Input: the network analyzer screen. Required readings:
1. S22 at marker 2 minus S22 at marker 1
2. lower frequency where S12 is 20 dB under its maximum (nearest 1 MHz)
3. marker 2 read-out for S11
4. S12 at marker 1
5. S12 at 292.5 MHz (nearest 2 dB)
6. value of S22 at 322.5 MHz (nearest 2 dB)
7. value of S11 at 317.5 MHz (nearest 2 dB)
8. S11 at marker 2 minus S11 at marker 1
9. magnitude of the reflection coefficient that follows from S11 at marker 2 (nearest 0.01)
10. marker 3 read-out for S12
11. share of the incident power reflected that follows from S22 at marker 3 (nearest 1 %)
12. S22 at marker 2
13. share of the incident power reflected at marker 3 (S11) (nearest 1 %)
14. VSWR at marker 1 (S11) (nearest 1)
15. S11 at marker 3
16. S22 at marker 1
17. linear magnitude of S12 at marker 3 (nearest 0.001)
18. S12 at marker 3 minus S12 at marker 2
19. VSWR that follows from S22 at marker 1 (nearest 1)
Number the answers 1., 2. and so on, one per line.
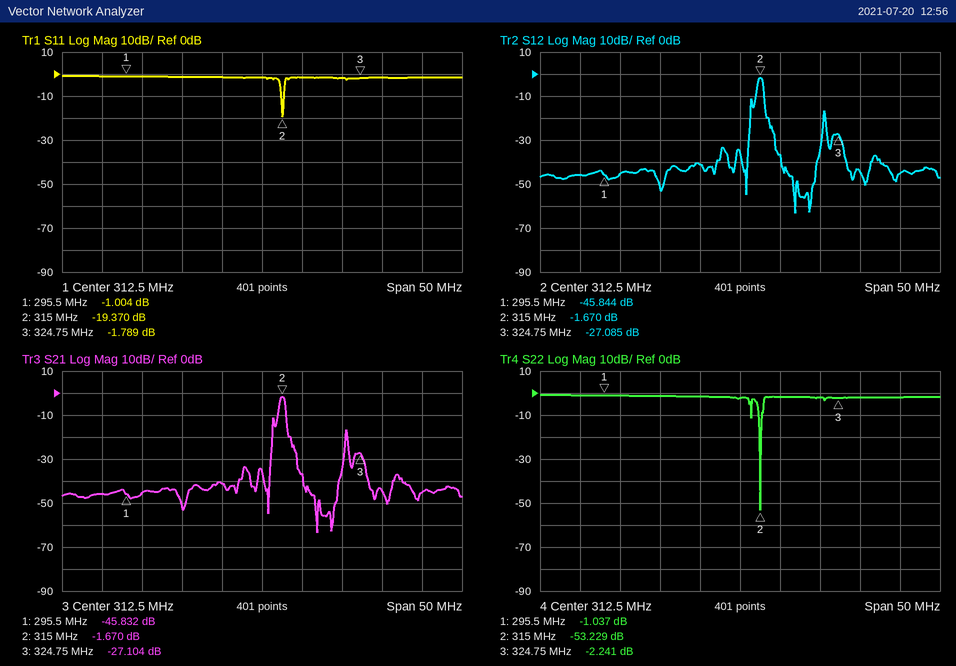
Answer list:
1. -52.192 dB
2. 314 MHz
3. -19.370 dB
4. -45.844 dB
5. -46 dB
6. -2 dB
7. -2 dB
8. -18.366 dB
9. 0.11
10. -27.085 dB
11. 60 %
12. -53.229 dB
13. 66 %
14. 17
15. -1.789 dB
16. -1.037 dB
17. 0.044
18. -25.415 dB
19. 17
